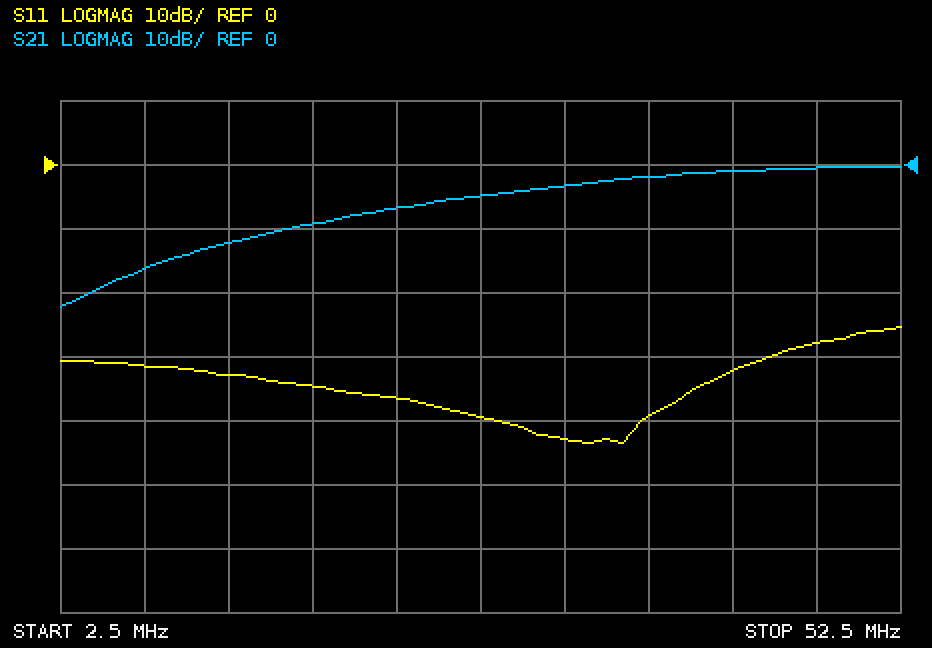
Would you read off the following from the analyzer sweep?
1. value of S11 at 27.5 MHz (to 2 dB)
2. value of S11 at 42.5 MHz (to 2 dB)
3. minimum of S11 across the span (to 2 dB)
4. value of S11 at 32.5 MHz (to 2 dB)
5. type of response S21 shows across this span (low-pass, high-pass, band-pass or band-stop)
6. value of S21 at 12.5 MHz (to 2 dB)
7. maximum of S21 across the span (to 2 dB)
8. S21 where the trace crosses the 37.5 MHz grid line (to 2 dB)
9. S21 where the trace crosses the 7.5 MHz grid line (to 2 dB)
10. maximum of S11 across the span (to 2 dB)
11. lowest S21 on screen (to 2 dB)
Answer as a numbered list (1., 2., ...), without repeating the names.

1. -40 dB
2. -32 dB
3. -44 dB
4. -42 dB
5. high-pass
6. -12 dB
7. 0 dB
8. -2 dB
9. -16 dB
10. -26 dB
11. -22 dB
